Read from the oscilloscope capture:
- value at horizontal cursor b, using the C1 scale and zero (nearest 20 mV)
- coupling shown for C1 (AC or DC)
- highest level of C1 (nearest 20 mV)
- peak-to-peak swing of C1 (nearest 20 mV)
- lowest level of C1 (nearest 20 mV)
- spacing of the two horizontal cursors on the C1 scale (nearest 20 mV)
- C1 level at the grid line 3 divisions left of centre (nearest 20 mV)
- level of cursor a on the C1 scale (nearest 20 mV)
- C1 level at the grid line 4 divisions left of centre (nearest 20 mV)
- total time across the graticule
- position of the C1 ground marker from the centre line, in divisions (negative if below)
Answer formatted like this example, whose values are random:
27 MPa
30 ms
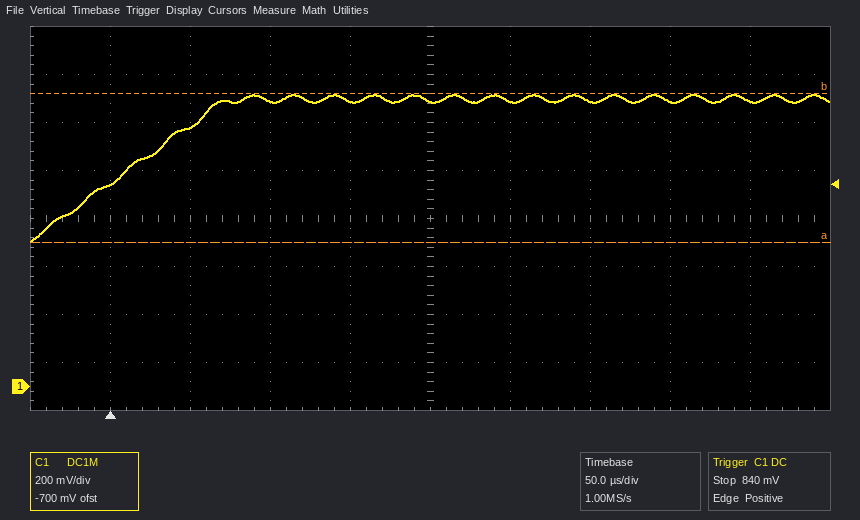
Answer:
1.22 V
DC
1.22 V
620 mV
600 mV
620 mV
1.08 V
600 mV
840 mV
500 µs
-3.5 div
